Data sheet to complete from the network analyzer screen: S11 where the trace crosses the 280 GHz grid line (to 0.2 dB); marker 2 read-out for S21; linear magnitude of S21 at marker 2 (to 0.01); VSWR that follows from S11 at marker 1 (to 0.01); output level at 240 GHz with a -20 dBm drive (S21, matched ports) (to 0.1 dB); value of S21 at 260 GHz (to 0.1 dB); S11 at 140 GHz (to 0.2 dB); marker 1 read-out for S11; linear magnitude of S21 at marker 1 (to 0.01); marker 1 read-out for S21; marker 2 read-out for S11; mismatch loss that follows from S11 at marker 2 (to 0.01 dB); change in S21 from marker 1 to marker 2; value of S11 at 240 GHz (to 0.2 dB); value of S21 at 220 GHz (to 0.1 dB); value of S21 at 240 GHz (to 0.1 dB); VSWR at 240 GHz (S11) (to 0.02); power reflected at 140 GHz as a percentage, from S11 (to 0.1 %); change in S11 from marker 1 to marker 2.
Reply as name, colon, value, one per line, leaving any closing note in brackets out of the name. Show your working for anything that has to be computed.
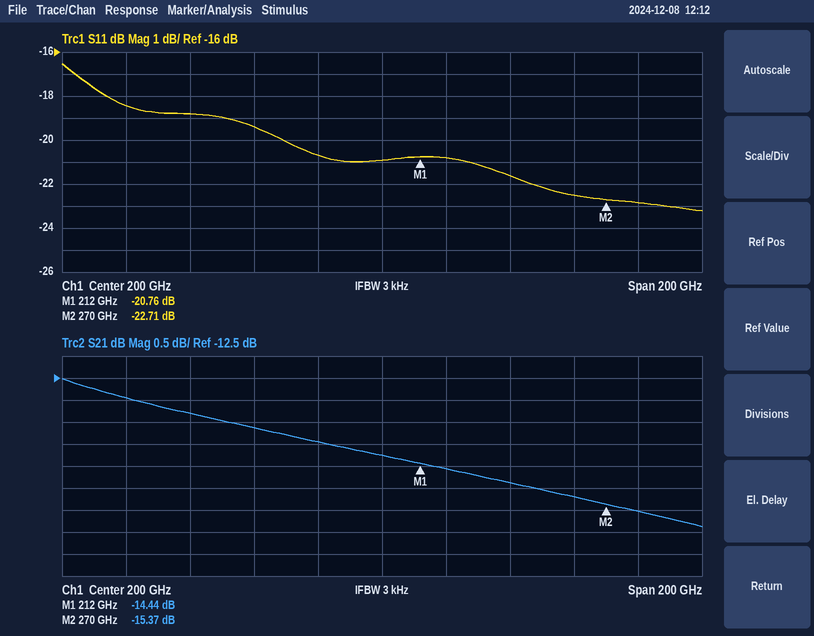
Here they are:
S11 where the trace crosses the 280 GHz grid line: -22.8 dB
marker 2 read-out for S21: -15.37 dB
linear magnitude of S21 at marker 2: 10^(-15.37/20) ≈ 0.17
VSWR that follows from S11 at marker 1: (1 + 0.0916)/(1 − 0.0916) ≈ 1.20
output level at 240 GHz with a -20 dBm drive (S21, matched ports): -20 dBm + (-14.9 dB) = -34.9 dBm
value of S21 at 260 GHz: -15.2 dB
S11 at 140 GHz: -18.8 dB
marker 1 read-out for S11: -20.76 dB
linear magnitude of S21 at marker 1: 10^(-14.44/20) ≈ 0.19
marker 1 read-out for S21: -14.44 dB
marker 2 read-out for S11: -22.71 dB
mismatch loss that follows from S11 at marker 2: −10 log10(1 − 10^(-22.71/10)) ≈ 0.02 dB
change in S21 from marker 1 to marker 2: -15.37 − (-14.44) = -0.93 dB
value of S11 at 240 GHz: -21.6 dB
value of S21 at 220 GHz: -14.6 dB
value of S21 at 240 GHz: -14.9 dB
VSWR at 240 GHz (S11): |Γ| = 10^(-21.6/20) = 0.0832; VSWR = (1 + 0.0832)/(1 − 0.0832) ≈ 1.18
power reflected at 140 GHz as a percentage, from S11: 10^(-18.8/10) ≈ 1.3 %
change in S11 from marker 1 to marker 2: -22.71 − (-20.76) = -1.95 dB
